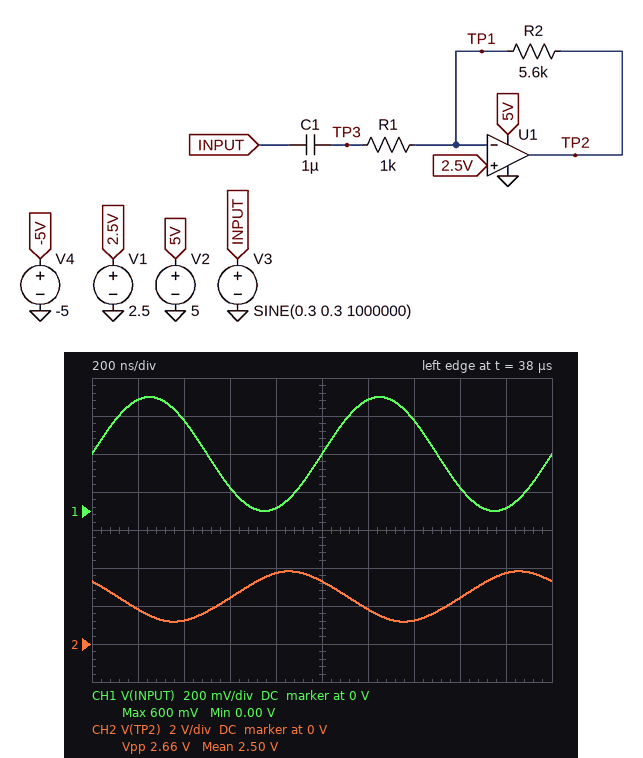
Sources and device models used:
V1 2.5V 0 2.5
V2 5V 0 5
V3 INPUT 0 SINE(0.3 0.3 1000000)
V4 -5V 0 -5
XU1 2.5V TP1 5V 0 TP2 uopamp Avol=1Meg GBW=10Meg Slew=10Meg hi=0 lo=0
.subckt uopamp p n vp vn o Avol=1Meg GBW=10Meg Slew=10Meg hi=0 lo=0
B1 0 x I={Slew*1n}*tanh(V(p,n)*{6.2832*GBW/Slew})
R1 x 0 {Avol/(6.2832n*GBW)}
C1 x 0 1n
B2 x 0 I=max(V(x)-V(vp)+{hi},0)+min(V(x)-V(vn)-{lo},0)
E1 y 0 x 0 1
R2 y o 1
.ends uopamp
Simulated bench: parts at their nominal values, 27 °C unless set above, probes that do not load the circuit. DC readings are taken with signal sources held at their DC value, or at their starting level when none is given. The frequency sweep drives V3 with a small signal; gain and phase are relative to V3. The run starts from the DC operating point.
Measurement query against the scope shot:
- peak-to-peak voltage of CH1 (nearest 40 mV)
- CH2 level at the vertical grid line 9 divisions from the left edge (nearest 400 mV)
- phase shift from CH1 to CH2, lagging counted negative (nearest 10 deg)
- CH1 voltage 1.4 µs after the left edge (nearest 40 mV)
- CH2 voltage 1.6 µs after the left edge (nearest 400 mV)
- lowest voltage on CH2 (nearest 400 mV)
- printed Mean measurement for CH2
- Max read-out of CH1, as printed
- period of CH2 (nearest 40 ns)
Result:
600 mV
3.6 V
140 deg
480 mV
2.4 V
1.2 V
2.50 V
600 mV
1.00 µs
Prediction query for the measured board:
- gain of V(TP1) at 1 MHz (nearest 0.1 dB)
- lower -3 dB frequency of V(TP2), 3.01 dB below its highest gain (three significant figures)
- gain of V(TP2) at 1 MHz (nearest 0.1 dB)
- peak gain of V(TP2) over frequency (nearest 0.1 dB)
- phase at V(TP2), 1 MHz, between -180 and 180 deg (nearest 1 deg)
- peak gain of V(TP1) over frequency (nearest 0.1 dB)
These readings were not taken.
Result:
-6.6 dB
159 Hz
13.4 dB
15.0 dB
147 deg
-1.4 dB
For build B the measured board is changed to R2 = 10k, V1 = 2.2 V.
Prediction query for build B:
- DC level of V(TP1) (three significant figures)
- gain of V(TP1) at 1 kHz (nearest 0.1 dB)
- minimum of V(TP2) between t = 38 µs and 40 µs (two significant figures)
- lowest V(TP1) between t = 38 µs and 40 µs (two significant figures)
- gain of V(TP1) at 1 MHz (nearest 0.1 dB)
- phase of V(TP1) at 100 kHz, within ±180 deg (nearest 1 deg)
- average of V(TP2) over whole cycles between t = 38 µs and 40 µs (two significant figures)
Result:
2.20 V
-60.1 dB
550 mV
2.0 V
-3.4 dB
84 deg
2.2 V
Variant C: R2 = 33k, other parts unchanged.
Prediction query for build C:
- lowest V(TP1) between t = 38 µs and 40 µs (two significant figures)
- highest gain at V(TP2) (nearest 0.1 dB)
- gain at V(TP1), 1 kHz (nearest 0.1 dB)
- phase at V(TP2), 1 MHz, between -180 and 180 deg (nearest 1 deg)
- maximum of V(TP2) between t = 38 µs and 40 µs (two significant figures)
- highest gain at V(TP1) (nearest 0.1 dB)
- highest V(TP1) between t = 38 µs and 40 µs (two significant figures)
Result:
2.2 V
30.4 dB
-49.7 dB
106 deg
4.3 V
-0.3 dB
2.8 V
